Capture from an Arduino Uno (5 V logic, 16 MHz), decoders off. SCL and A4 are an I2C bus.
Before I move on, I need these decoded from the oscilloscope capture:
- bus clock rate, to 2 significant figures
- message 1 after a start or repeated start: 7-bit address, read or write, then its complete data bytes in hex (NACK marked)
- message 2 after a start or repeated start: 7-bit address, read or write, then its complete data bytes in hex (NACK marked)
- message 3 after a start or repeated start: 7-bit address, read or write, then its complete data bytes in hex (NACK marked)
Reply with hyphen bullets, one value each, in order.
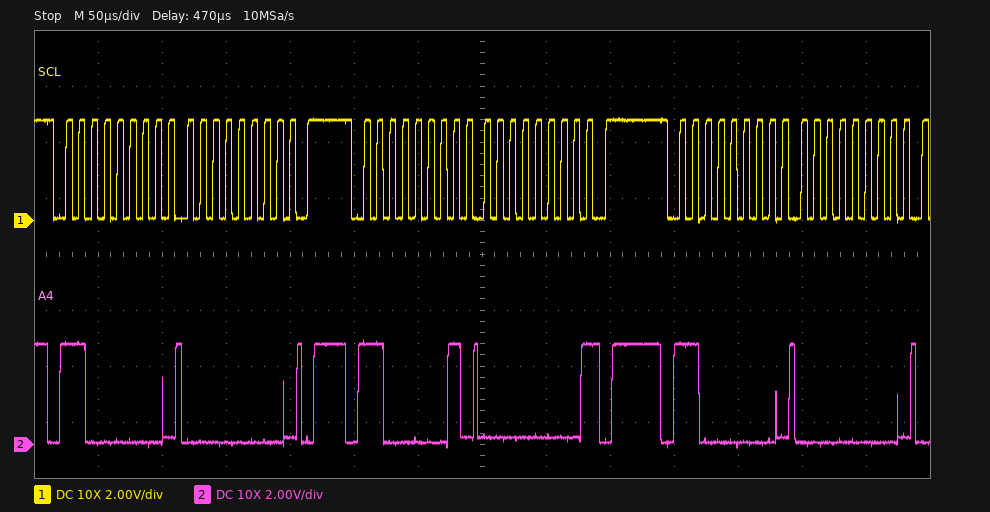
- 100 kHz
- 0x60 write: 00
- 0x60 read: 00 NACK
- 0x60 write: 00
